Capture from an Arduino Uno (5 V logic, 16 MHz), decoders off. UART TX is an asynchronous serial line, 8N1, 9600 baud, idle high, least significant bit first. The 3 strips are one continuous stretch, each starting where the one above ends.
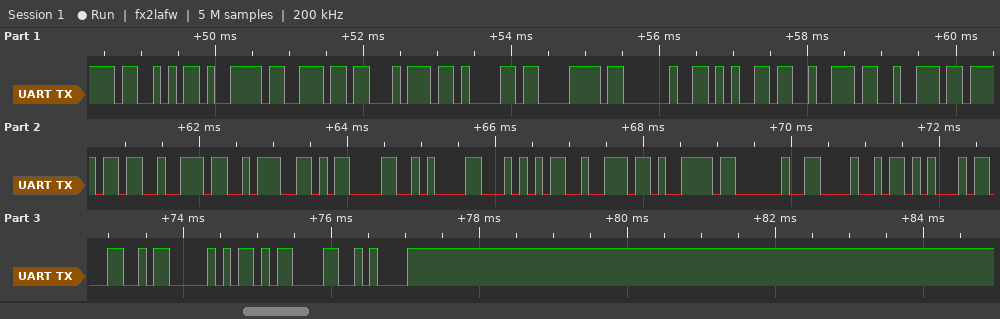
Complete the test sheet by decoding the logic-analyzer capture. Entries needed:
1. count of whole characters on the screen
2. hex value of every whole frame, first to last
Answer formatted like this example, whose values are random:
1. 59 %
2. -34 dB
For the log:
1. 25
2. 53 79 6E 74 61 78 20 65 72 72 6F 72 3A 0D 0A 54 72 79 20 48 45 4C 50 0D 0A
